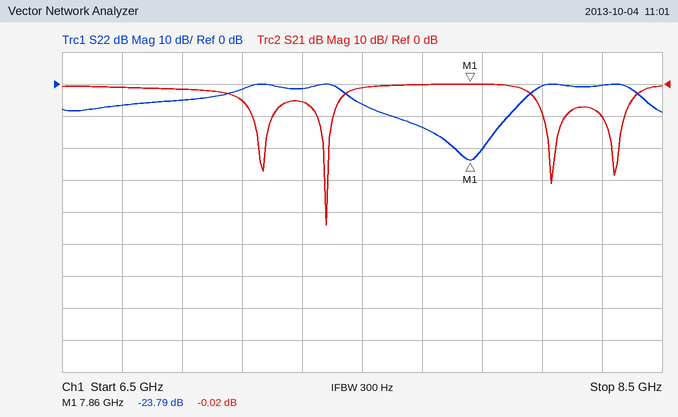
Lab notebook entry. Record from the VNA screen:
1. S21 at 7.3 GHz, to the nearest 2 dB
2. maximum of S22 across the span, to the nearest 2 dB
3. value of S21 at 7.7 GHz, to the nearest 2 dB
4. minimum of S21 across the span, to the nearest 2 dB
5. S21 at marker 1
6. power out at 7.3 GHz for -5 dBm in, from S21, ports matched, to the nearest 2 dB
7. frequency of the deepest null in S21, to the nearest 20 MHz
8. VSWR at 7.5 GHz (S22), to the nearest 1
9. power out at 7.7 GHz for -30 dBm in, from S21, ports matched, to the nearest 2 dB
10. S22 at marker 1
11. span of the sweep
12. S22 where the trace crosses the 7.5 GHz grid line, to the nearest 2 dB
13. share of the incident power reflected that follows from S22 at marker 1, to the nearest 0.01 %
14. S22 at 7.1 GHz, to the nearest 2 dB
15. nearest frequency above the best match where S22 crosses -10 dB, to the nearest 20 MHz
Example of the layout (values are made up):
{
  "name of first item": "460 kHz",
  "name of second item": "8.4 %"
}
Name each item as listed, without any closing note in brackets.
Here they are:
{
  "S21 at 7.3 GHz, to the nearest 2 dB": "-6 dB",
  "maximum of S22 across the span, to the nearest 2 dB": "0 dB",
  "value of S21 at 7.7 GHz, to the nearest 2 dB": "0 dB",
  "minimum of S21 across the span, to the nearest 2 dB": "-44 dB",
  "S21 at marker 1": "-0.02 dB",
  "power out at 7.3 GHz for -5 dBm in, from S21, ports matched, to the nearest 2 dB": "-10 dBm",
  "frequency of the deepest null in S21, to the nearest 20 MHz": "7.38 GHz",
  "VSWR at 7.5 GHz (S22), to the nearest 1": "3",
  "power out at 7.7 GHz for -30 dBm in, from S21, ports matched, to the nearest 2 dB": "-30 dBm",
  "S22 at marker 1": "-23.79 dB",
  "span of the sweep": "2 GHz",
  "S22 where the trace crosses the 7.5 GHz grid line, to the nearest 2 dB": "-6 dB",
  "share of the incident power reflected that follows from S22 at marker 1, to the nearest 0.01 %": "0.42 %",
  "S22 at 7.1 GHz, to the nearest 2 dB": "-2 dB",
  "nearest frequency above the best match where S22 crosses -10 dB, to the nearest 20 MHz": "7.98 GHz"
}
